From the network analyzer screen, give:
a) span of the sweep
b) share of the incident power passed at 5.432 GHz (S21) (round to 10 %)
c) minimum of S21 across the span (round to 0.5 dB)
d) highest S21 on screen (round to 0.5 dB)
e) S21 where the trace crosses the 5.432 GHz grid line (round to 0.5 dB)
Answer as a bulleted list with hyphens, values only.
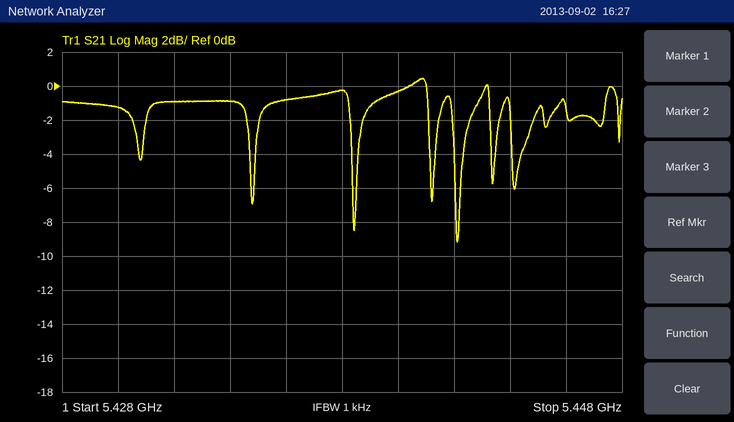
- 20 MHz
- 80 %
- -9.0 dB
- 0.5 dB
- -1.0 dB
